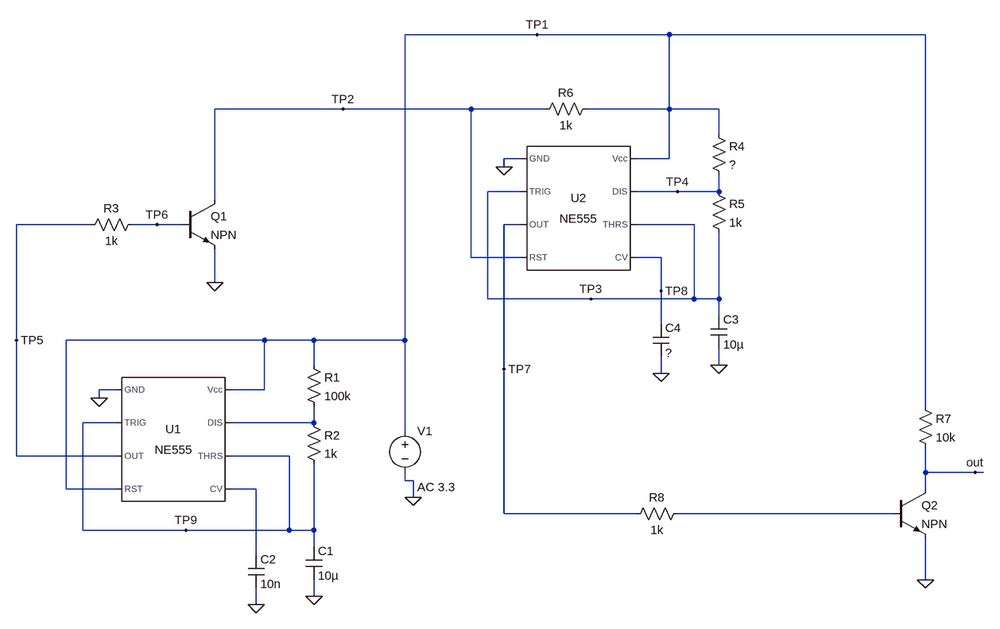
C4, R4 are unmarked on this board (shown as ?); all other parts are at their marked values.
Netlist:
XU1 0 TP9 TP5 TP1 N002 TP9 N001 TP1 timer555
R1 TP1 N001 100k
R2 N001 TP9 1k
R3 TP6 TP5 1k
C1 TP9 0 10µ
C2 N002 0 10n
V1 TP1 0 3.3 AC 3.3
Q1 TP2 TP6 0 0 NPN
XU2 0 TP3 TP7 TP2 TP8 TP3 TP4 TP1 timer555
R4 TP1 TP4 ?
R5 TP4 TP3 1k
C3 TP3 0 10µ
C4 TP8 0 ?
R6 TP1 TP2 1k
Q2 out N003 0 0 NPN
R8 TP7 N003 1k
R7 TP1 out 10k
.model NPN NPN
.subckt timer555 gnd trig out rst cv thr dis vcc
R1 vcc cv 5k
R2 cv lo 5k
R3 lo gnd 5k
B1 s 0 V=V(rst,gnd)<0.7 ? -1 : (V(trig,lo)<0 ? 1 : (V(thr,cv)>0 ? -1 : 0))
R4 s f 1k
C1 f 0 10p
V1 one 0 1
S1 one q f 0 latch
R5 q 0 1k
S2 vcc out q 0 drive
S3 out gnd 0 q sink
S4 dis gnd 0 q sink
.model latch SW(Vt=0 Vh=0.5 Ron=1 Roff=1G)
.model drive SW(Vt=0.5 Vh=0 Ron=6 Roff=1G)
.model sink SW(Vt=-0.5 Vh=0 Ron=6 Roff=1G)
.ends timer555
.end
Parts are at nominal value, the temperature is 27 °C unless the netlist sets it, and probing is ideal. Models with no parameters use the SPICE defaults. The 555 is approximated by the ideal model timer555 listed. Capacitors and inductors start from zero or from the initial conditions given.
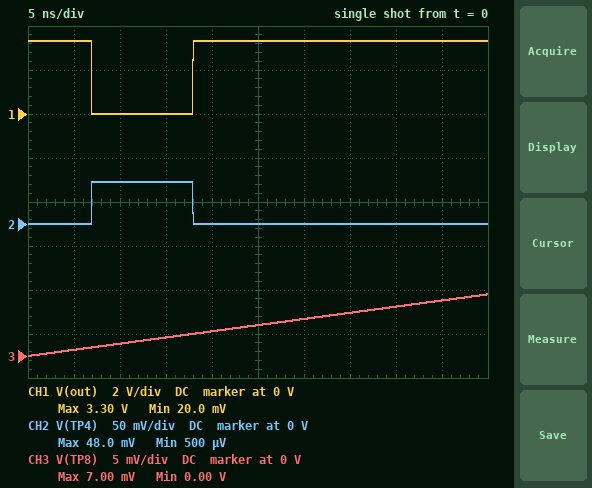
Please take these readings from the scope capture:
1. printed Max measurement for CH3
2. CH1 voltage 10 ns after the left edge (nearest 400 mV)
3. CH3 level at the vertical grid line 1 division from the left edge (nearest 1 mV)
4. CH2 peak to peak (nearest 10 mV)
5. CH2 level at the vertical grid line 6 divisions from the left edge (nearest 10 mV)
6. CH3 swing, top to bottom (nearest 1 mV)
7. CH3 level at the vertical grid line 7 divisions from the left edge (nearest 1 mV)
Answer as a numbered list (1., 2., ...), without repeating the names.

1. 7.00 mV
2. 0 V
3. 1 mV
4. 50 mV
5. 0 V
6. 7 mV
7. 5 mV
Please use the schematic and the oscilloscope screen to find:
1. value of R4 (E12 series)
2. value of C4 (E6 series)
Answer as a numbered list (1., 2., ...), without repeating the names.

1. 68 kΩ
2. 4.7 nF
